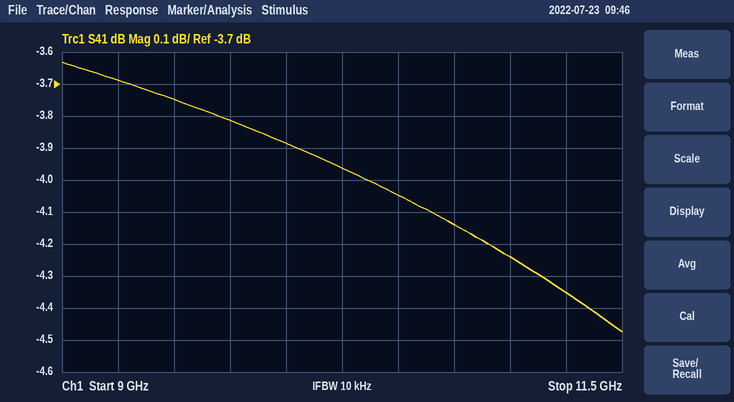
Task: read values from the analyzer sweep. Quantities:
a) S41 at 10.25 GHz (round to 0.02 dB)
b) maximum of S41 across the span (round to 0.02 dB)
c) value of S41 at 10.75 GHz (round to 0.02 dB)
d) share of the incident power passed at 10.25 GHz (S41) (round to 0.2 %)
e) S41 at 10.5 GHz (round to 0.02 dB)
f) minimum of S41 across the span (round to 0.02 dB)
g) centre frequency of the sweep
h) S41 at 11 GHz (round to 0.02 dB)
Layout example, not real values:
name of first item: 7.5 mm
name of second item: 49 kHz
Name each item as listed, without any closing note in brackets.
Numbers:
S41 at 10.25 GHz: -3.96 dB
maximum of S41 across the span: -3.64 dB
value of S41 at 10.75 GHz: -4.14 dB
share of the incident power passed at 10.25 GHz (S41): 40.2 %
S41 at 10.5 GHz: -4.04 dB
minimum of S41 across the span: -4.48 dB
centre frequency of the sweep: 10.25 GHz
S41 at 11 GHz: -4.24 dB
